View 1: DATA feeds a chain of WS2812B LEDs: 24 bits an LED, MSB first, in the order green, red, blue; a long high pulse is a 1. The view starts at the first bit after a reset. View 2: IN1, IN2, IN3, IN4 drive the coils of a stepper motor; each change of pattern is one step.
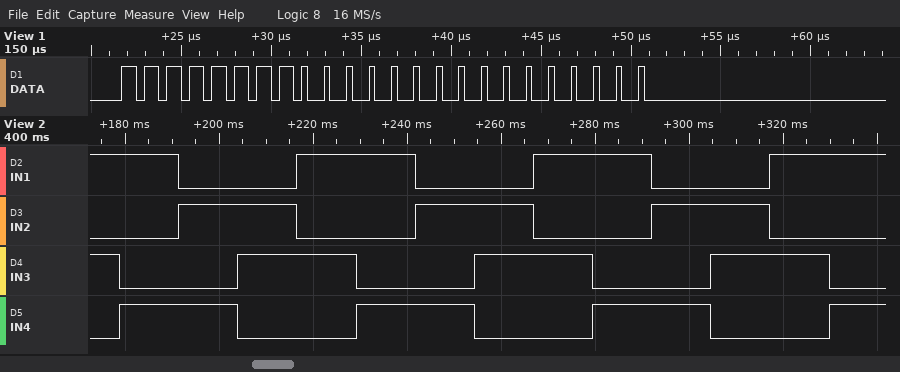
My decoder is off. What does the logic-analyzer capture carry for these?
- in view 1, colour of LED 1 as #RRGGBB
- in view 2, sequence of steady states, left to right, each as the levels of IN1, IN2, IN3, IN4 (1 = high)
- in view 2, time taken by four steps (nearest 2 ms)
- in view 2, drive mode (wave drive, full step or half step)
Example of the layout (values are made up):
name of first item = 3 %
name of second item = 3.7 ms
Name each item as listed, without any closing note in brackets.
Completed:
in view 1, colour of LED 1 as #RRGGBB = #00FF00
in view 2, sequence of steady states, left to right, each as the levels of IN1, IN2, IN3, IN4 = 1010 1001 0101 0110 1010 1001 0101 0110 1010 1001 0101 0110 1010 1001
in view 2, time taken by four steps = 50 ms
in view 2, drive mode = full step
